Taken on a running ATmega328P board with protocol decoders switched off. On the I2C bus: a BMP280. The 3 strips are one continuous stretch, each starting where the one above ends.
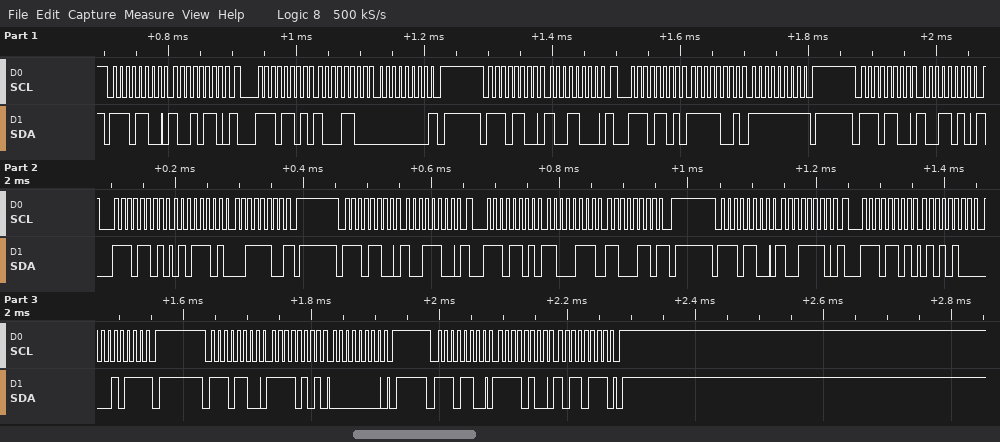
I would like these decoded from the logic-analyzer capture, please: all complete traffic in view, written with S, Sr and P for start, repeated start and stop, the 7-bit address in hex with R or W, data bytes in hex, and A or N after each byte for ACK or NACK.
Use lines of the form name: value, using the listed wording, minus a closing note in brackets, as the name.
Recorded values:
all complete traffic in view, written with S, Sr and P for start, repeated start and stop, the 7-bit address in hex with R or W, data bytes in hex, and A or N after each byte for ACK or NACK: S 76W A 96 A Sr 76R A 8C A 00 N P S 76W A 98 A Sr 76R A F9 A FF N P S 76W A 9A A Sr 76R A 5D A 3C N P S 76W A 9C A Sr 76R A C7 A C6 N P S 76W A 9E A Sr 76R A 54 A 17 N P S 76W A F5 A 00 A P S 76W A F4 A B7 A P
